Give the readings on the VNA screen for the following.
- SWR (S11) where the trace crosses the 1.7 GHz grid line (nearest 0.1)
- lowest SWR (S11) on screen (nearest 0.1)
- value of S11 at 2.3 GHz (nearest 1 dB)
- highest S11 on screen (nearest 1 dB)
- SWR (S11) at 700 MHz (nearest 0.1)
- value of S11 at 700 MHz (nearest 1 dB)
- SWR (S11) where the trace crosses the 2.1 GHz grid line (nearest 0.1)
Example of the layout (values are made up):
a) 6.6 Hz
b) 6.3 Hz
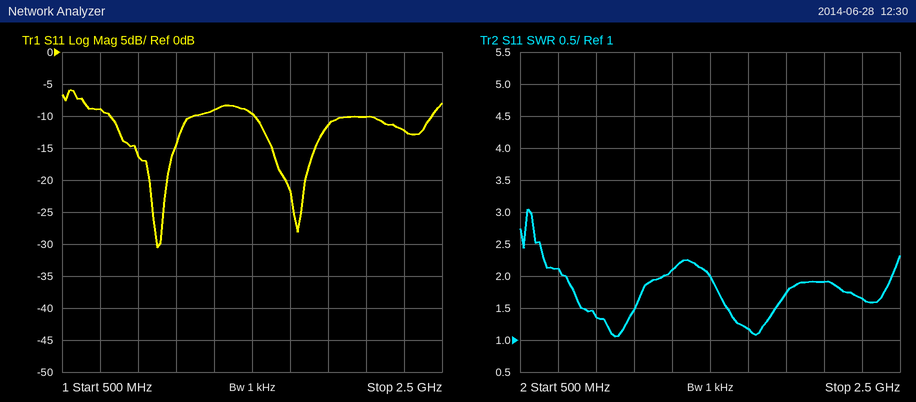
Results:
a) 1.2
b) 1.1
c) -12 dB
d) -6 dB
e) 2.1
f) -9 dB
g) 1.9
